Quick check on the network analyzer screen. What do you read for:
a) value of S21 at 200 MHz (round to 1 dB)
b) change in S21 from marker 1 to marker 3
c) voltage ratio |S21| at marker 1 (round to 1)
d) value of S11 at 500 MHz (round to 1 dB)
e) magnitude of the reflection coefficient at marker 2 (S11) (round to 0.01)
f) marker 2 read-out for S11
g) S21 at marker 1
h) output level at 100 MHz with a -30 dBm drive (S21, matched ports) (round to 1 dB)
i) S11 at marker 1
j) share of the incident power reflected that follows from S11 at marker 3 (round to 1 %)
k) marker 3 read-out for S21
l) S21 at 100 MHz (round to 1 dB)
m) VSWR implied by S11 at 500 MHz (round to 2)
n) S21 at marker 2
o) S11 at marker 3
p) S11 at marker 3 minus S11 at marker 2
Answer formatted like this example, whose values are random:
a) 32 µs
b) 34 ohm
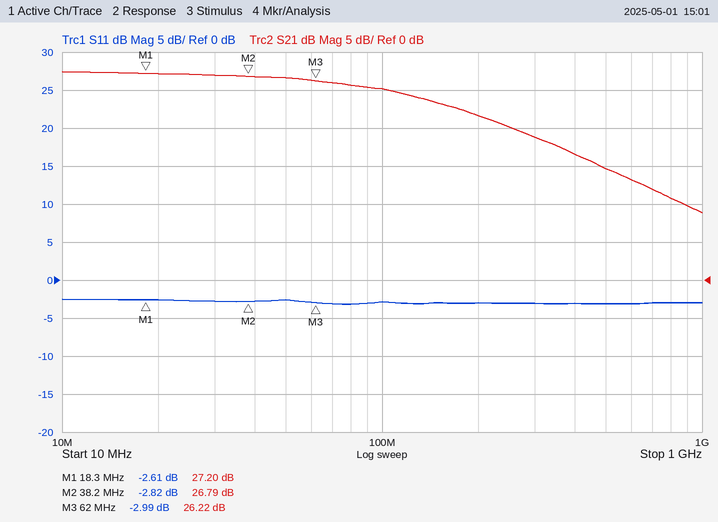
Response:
a) 22 dB
b) -0.98 dB
c) 23
d) -3 dB
e) 0.72
f) -2.82 dB
g) 27.20 dB
h) -5 dBm
i) -2.61 dB
j) 50 %
k) 26.22 dB
l) 25 dB
m) 6
n) 26.79 dB
o) -2.99 dB
p) -0.17 dB
